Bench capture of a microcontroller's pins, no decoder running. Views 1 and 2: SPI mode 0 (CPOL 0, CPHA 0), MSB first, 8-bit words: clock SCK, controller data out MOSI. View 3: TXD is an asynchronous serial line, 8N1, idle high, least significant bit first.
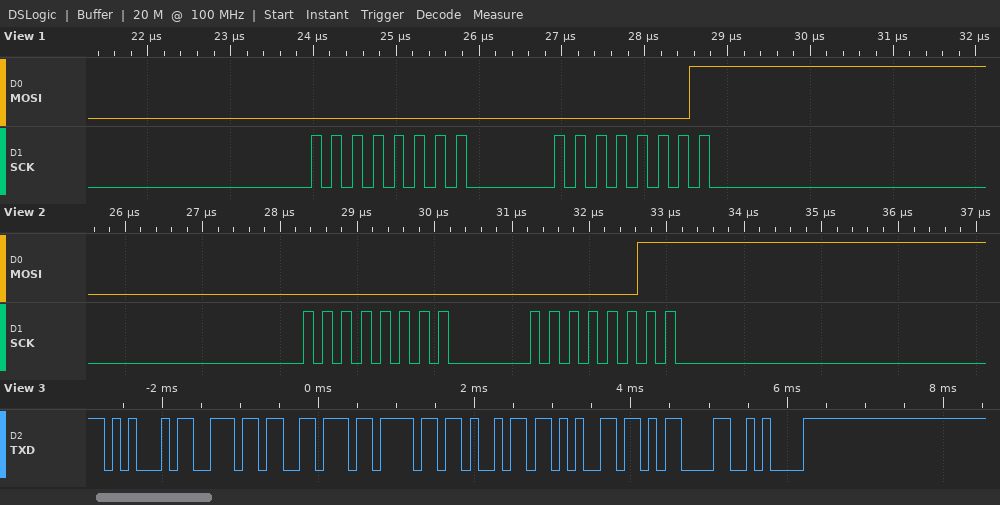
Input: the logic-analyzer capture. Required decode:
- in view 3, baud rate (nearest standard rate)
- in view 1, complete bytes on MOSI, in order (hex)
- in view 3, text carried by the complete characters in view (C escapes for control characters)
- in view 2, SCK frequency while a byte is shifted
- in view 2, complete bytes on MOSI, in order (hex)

9600 baud
00 01
"Envoie\r\n"
4 MHz
0x00 0x03
